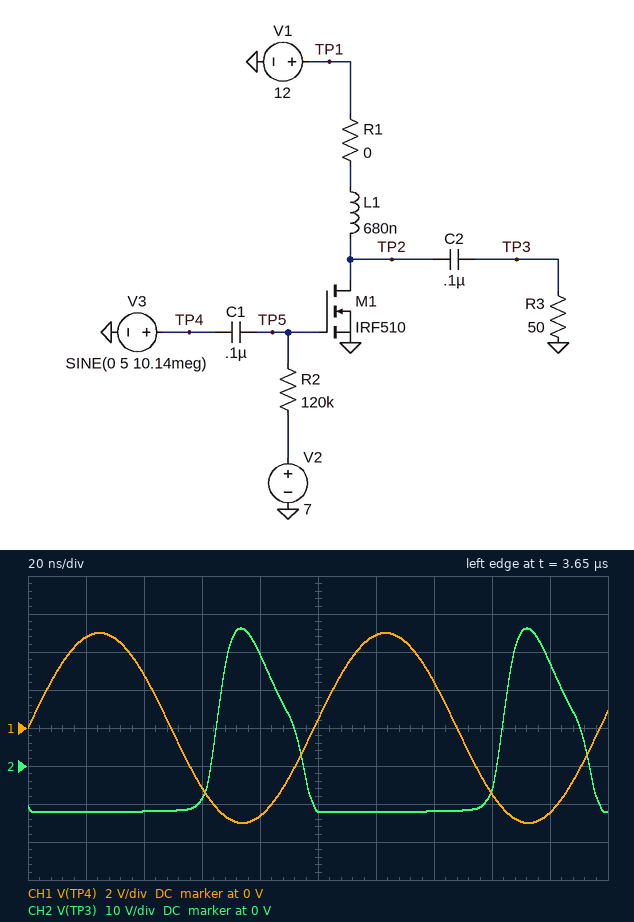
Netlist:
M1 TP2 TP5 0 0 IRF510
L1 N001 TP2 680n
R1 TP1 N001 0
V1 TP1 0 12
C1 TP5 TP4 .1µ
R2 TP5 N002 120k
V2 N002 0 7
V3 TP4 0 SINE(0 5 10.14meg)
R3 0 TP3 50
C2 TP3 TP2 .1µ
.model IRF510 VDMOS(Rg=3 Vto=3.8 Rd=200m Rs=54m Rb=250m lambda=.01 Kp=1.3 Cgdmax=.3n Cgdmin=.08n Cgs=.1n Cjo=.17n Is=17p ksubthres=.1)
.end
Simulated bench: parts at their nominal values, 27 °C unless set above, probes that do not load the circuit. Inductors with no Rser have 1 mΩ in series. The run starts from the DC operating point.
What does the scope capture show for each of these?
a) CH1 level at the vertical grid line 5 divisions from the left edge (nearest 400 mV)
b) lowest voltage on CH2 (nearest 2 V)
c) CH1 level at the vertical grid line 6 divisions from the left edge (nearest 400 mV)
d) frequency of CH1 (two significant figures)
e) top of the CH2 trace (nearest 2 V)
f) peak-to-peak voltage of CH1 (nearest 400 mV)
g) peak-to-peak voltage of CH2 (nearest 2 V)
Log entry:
400 mV
-12 V
4.8 V
10 MHz
36 V
10.0 V
48 V
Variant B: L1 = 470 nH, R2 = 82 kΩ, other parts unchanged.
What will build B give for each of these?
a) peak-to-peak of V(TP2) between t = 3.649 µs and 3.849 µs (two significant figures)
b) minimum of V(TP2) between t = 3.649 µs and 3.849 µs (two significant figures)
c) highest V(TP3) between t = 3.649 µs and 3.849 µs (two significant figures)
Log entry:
55 V
170 mV
43 V
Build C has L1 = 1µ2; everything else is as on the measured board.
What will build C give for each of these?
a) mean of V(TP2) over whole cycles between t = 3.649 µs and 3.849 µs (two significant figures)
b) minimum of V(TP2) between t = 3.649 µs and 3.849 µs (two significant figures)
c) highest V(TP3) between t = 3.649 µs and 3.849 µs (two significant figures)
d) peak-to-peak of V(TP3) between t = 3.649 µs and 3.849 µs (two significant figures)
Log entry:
12 V
240 mV
30 V
43 V
